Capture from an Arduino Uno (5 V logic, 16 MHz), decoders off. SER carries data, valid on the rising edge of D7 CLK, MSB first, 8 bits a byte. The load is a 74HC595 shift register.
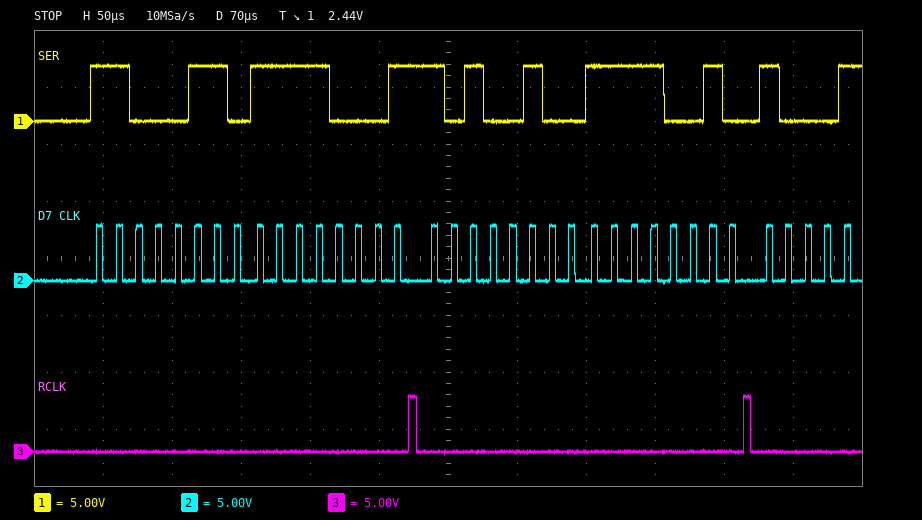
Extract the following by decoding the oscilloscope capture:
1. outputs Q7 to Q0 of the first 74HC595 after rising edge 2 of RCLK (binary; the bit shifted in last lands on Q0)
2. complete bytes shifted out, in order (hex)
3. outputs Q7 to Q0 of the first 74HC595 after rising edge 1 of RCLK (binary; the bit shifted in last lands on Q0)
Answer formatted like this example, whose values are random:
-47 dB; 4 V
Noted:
11110010; 0xC6 0xF1 0xA4 0xF2; 11110001
